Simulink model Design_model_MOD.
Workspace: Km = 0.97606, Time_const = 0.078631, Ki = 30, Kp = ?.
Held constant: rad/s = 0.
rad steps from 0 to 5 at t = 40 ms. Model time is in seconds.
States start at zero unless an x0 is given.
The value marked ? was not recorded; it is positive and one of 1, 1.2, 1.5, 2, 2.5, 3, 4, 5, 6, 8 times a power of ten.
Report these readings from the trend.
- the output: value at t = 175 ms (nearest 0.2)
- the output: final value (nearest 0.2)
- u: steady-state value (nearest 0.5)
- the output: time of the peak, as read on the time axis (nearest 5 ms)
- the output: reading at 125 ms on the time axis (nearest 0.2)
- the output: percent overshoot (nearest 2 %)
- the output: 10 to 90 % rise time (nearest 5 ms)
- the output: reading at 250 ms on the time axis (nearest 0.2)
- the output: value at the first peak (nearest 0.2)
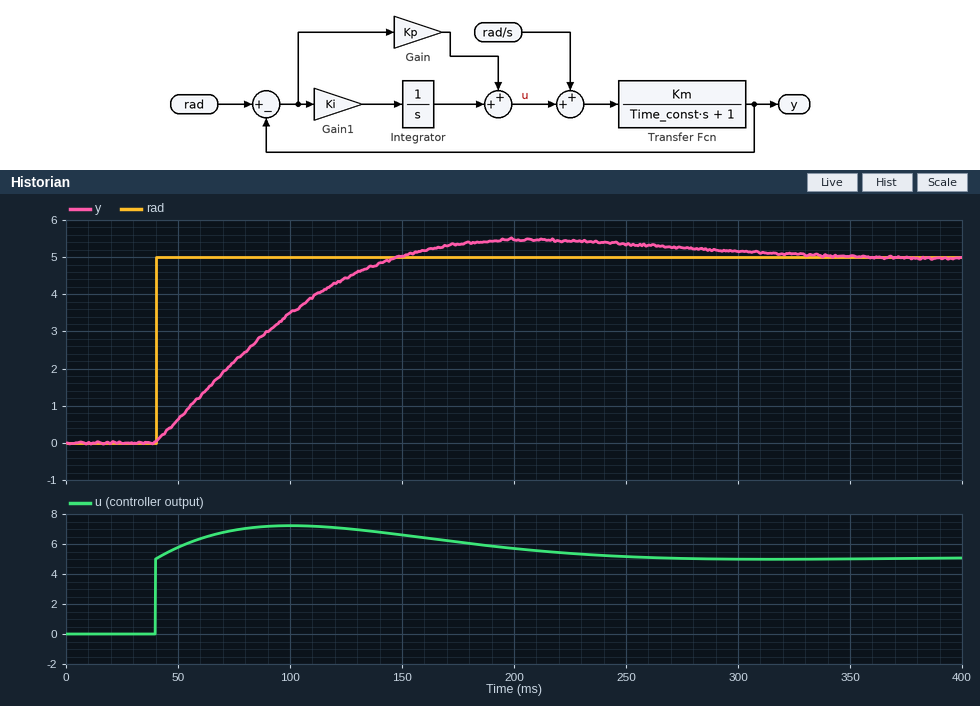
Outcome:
5.4
5.0
5.0
205 ms
4.4
10 %
80 ms
5.4
5.4
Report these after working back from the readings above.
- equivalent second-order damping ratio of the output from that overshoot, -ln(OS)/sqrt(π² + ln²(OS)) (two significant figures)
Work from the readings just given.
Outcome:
0.59
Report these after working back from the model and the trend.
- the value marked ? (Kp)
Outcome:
1
